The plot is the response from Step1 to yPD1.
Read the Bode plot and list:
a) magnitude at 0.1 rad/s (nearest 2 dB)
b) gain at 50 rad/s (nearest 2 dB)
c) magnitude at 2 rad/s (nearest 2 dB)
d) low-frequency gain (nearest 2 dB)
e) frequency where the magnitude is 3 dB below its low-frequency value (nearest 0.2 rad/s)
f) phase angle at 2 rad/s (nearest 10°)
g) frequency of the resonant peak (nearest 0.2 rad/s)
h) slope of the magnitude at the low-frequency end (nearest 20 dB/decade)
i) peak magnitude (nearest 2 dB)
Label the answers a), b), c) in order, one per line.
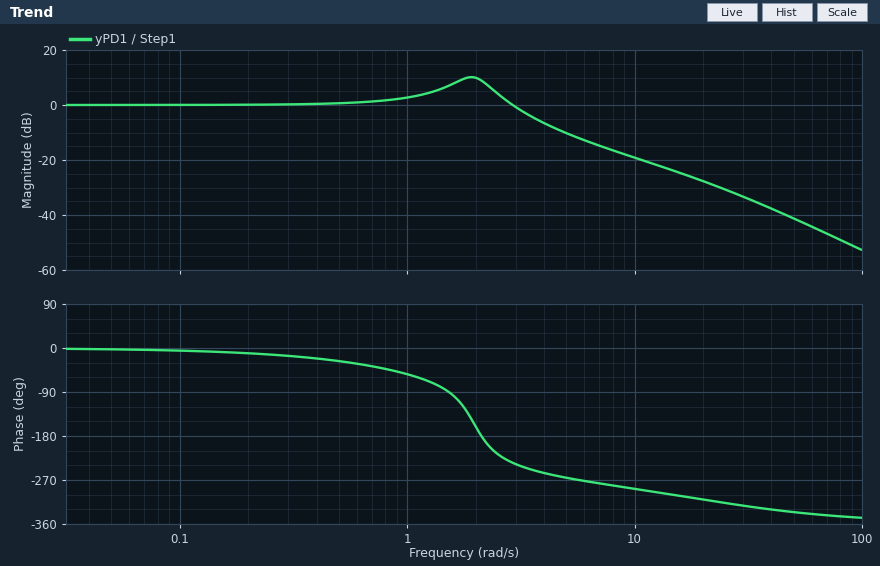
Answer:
a) 0 dB
b) -42 dB
c) 10 dB
d) 0 dB
e) 3.4 rad/s
f) -160°
g) 2.0 rad/s
h) 0 dB/decade
i) 10 dB
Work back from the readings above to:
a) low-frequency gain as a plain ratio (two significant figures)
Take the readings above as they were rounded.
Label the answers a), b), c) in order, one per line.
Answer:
a) 1.0
